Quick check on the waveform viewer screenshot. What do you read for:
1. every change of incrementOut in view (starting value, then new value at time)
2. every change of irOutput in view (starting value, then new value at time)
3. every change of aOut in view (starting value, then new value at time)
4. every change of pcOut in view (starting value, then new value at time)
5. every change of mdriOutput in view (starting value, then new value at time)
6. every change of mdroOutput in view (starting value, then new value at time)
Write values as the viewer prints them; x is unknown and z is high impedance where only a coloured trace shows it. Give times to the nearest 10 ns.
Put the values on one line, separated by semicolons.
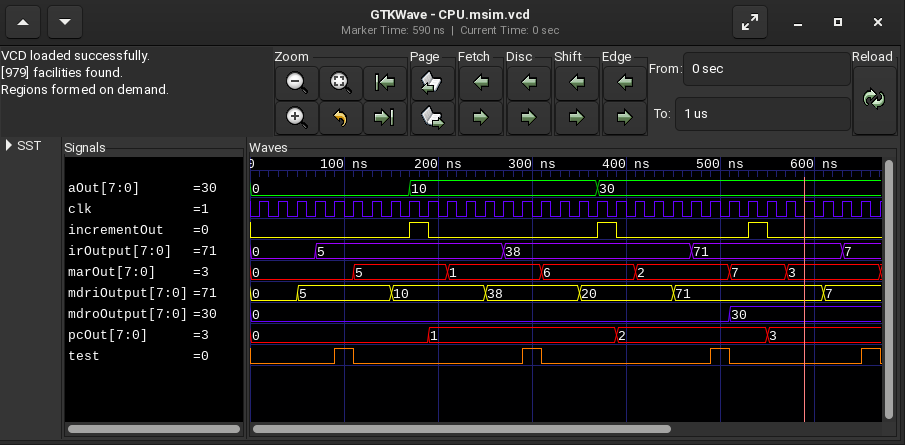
0, 1 at 170 ns, 0 at 190 ns, 1 at 370 ns, 0 at 390 ns, 1 at 530 ns, 0 at 550 ns; 0, 5 at 70 ns, 38 at 270 ns, 71 at 470 ns, 7 at 630 ns; 0, 10 at 170 ns, 30 at 370 ns; 0, 1 at 190 ns, 2 at 390 ns, 3 at 550 ns; 0, 5 at 50 ns, 10 at 150 ns, 38 at 250 ns, 20 at 350 ns, 71 at 450 ns, 7 at 610 ns; 0, 30 at 510 ns
